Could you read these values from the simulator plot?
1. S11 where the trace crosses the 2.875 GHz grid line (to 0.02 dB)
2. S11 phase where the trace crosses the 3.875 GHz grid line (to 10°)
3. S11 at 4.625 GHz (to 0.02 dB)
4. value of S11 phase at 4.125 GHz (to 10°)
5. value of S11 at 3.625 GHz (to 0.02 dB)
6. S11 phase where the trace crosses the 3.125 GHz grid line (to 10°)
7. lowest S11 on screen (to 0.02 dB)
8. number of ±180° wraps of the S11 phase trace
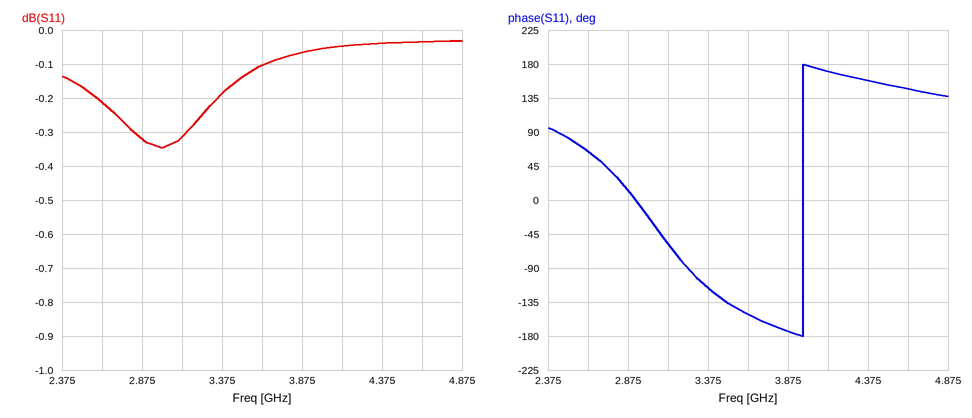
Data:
-0.32 dB
-170°
-0.04 dB
170°
-0.10 dB
-60°
-0.34 dB
1
